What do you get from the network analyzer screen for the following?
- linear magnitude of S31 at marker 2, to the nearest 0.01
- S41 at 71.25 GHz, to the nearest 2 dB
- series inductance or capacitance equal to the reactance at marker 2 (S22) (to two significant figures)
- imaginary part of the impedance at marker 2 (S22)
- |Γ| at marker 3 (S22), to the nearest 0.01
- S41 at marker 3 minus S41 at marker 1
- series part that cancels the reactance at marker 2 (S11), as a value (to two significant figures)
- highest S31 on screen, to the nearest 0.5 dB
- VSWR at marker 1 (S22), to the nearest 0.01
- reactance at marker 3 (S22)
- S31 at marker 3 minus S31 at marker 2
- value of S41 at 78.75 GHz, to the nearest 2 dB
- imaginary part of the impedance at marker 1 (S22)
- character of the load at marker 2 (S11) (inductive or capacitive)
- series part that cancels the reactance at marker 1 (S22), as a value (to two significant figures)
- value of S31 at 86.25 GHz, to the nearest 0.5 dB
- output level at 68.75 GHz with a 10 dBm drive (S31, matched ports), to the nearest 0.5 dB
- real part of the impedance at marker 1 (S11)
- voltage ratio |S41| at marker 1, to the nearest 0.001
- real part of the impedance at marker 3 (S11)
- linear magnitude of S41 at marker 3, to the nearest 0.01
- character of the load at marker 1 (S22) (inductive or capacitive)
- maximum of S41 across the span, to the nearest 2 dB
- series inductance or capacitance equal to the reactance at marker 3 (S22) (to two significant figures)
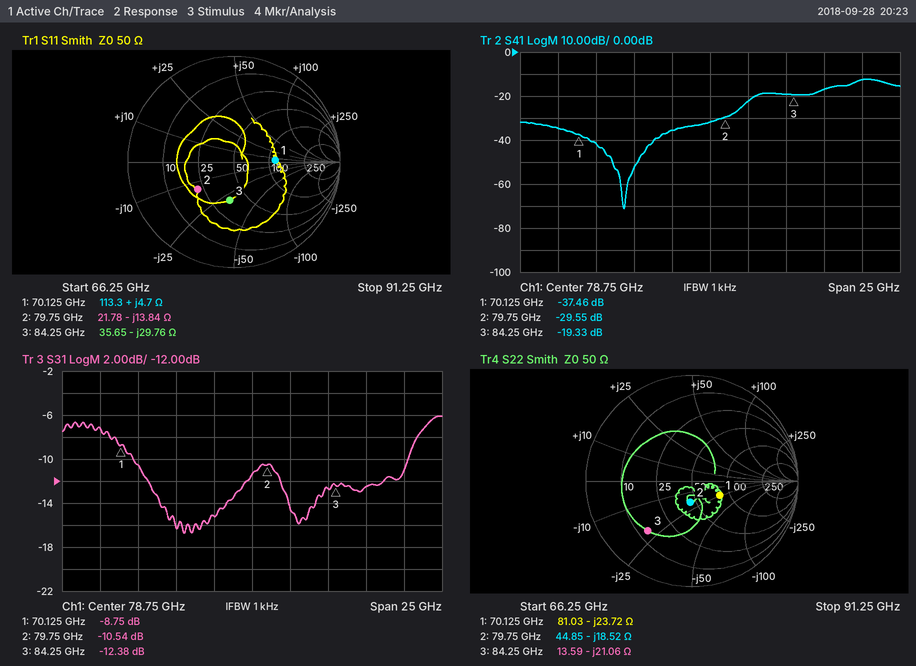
0.30
-42 dB
110 fF
-18.52 Ω
0.63
18.13 dB
28 pH
-6.0 dB
1.83
-21.06 Ω
-1.84 dB
-32 dB
-23.72 Ω
capacitive
54 pH
-12.5 dB
3.0 dBm
113.3 Ω
0.013
35.65 Ω
0.11
capacitive
-12 dB
90 fF
